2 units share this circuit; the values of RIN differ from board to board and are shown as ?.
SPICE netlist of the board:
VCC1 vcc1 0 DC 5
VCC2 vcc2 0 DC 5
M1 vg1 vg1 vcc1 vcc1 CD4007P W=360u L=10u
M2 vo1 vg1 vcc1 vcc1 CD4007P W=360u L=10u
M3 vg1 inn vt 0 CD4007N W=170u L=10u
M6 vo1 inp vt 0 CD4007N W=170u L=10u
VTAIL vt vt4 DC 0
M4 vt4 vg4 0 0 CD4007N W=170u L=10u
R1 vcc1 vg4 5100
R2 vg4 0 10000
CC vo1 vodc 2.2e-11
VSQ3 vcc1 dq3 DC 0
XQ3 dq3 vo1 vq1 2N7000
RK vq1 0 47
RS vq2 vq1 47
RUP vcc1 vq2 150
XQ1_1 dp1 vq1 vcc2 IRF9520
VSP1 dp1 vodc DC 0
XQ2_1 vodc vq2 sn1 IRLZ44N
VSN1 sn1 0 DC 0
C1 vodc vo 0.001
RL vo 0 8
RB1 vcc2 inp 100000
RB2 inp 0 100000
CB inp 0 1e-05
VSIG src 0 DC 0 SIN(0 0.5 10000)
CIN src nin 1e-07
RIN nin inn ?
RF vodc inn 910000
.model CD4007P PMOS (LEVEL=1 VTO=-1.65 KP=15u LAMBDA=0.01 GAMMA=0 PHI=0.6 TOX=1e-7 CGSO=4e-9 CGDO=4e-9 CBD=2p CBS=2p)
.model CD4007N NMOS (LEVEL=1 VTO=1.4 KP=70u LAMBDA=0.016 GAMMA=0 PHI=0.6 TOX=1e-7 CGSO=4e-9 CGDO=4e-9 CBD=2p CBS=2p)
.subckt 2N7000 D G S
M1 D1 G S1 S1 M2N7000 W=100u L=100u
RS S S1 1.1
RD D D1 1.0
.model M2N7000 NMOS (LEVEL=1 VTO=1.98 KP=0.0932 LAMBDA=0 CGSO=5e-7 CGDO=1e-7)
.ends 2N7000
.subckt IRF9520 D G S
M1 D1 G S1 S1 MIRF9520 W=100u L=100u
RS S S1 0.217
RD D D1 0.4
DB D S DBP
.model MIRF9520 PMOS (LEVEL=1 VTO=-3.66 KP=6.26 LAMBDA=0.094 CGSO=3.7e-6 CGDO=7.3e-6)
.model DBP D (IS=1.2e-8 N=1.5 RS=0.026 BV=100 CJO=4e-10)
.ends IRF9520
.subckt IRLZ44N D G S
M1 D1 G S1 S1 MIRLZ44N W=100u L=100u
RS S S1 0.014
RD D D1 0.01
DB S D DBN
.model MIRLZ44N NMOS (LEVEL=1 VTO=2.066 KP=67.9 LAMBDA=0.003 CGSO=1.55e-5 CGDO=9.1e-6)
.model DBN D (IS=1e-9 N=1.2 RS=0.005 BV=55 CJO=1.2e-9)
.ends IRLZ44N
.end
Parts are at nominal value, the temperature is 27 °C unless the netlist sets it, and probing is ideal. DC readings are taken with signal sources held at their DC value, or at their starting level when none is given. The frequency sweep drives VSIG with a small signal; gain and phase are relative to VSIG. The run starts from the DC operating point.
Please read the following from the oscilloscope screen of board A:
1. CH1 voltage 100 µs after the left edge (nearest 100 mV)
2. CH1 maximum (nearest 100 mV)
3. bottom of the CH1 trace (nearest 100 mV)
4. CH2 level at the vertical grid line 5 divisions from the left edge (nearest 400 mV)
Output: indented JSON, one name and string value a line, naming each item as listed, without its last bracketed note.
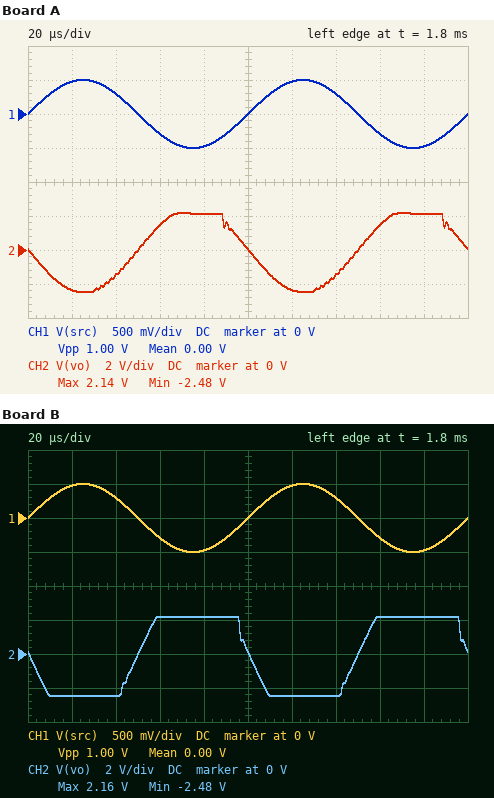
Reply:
{
  "CH1 voltage 100 µs after the left edge": "0 V",
  "CH1 maximum": "500 mV",
  "bottom of the CH1 trace": "-500 mV",
  "CH2 level at the vertical grid line 5 divisions from the left edge": "0 V"
}
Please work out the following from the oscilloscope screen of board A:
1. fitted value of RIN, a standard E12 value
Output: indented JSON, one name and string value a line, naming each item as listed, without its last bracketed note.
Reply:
{
  "fitted value of RIN, a standard E12 value": "180 kΩ"
}
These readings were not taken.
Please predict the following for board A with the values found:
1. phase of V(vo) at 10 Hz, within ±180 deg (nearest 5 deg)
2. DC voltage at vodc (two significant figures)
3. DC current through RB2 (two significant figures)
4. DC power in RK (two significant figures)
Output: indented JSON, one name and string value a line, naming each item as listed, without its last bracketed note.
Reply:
{
  "phase of V(vo) at 10 Hz, within ±180 deg": "-75 deg",
  "DC voltage at vodc": "2.5 V",
  "DC current through RB2": "25 µA",
  "DC power in RK": "31 mW"
}
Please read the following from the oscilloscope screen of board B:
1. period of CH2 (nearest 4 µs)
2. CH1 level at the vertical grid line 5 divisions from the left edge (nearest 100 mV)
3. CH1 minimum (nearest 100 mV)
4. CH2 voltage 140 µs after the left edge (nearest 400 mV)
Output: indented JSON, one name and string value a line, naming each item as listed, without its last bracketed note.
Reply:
{
  "period of CH2": "100 µs",
  "CH1 level at the vertical grid line 5 divisions from the left edge": "0 V",
  "CH1 minimum": "-500 mV",
  "CH2 voltage 140 µs after the left edge": "-2.4 V"
}
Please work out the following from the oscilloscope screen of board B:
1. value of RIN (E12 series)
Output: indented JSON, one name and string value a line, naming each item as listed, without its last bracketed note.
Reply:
{
  "value of RIN": "100 kΩ"
}
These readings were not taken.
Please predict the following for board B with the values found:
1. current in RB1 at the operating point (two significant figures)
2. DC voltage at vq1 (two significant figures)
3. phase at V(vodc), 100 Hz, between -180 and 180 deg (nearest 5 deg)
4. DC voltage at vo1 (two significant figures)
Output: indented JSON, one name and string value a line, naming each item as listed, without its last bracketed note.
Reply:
{
  "current in RB1 at the operating point": "25 µA",
  "DC voltage at vq1": "1.2 V",
  "phase at V(vodc), 100 Hz, between -180 and 180 deg": "-170 deg",
  "DC voltage at vo1": "3.6 V"
}
